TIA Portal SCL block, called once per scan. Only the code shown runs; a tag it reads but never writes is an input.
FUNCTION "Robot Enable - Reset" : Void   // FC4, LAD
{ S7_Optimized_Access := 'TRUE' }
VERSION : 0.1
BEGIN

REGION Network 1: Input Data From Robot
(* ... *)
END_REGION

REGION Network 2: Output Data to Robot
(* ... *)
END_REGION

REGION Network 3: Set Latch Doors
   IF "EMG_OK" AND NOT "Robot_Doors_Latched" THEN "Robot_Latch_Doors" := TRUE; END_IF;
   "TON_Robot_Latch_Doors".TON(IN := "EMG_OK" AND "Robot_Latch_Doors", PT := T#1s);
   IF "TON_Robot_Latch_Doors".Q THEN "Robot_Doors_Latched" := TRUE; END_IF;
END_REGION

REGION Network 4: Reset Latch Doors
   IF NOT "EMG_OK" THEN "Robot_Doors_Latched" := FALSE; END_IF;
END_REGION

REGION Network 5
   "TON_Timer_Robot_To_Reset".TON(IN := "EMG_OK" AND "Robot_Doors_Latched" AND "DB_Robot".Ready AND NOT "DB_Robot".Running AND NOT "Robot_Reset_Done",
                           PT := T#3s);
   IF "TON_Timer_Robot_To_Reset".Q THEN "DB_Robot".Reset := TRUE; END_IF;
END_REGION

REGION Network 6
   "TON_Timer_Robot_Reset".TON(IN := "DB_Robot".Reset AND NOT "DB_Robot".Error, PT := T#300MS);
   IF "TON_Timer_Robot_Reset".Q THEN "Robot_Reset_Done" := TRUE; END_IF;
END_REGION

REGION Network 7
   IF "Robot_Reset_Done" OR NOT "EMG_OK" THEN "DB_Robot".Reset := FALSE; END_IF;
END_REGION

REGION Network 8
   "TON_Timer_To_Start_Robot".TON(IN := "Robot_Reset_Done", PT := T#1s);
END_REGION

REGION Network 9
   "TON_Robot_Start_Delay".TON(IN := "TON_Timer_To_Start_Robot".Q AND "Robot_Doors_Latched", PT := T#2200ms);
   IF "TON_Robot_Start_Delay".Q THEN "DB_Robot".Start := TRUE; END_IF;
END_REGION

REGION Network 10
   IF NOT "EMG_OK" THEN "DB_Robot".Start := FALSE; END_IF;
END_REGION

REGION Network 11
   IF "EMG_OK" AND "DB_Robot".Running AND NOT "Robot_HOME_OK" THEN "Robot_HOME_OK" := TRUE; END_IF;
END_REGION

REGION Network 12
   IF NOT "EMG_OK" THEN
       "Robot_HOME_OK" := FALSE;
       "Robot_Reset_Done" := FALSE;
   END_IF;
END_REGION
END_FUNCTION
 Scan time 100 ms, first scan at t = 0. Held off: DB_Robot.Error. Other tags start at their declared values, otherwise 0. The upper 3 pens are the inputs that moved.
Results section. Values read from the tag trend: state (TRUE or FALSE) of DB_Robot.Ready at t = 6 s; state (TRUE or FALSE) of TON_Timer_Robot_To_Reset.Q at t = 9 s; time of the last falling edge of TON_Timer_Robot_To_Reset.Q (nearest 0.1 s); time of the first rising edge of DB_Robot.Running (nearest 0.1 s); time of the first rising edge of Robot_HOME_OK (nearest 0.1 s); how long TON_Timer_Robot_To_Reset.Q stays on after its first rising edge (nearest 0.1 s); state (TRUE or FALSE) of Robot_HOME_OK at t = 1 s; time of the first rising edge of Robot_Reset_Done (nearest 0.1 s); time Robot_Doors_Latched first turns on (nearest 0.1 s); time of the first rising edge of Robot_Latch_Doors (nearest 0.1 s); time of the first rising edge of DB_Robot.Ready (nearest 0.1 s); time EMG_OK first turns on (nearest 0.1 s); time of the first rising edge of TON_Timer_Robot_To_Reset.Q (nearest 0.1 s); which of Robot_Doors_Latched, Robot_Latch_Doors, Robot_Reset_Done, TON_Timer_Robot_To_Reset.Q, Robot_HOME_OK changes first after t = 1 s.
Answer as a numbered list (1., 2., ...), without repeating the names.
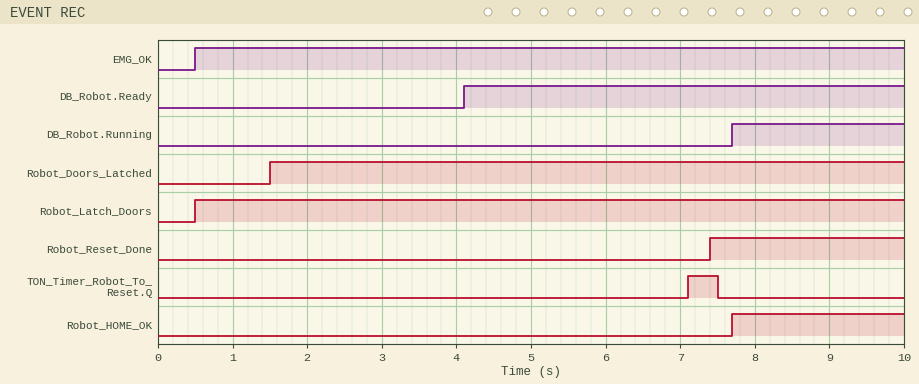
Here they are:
1. TRUE
2. FALSE
3. 7.5 s
4. 7.7 s
5. 7.7 s
6. 0.4 s
7. FALSE
8. 7.4 s
9. 1.5 s
10. 0.5 s
11. 4.1 s
12. 0.5 s
13. 7.1 s
14. Robot_Doors_Latched
